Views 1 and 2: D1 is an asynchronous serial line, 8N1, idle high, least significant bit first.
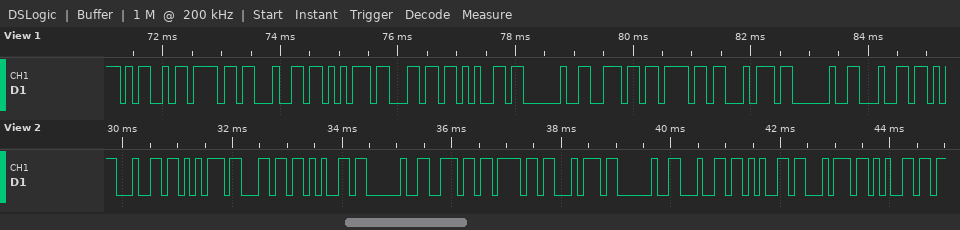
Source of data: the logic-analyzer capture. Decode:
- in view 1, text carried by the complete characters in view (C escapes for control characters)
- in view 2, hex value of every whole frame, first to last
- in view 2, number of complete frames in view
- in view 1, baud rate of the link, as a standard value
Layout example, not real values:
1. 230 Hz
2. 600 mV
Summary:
1. "Module not d"
2. 64 75 6C 65 20 6E 6F 74 20 64 65 74 65
3. 13
4. 9600 baud
